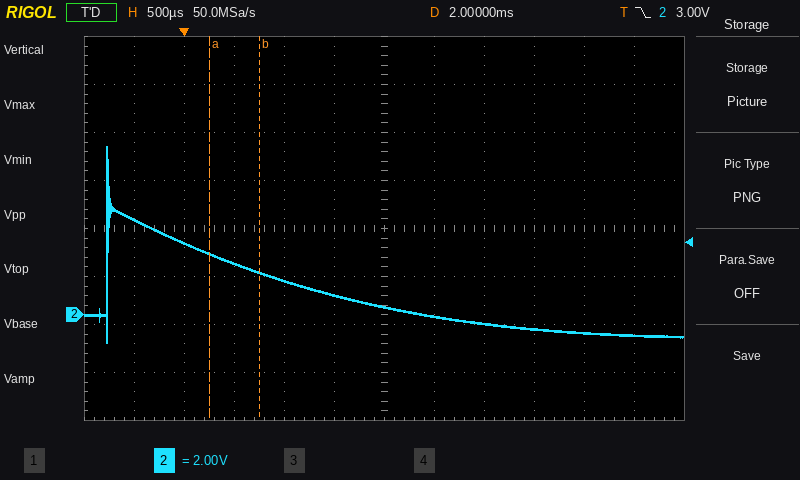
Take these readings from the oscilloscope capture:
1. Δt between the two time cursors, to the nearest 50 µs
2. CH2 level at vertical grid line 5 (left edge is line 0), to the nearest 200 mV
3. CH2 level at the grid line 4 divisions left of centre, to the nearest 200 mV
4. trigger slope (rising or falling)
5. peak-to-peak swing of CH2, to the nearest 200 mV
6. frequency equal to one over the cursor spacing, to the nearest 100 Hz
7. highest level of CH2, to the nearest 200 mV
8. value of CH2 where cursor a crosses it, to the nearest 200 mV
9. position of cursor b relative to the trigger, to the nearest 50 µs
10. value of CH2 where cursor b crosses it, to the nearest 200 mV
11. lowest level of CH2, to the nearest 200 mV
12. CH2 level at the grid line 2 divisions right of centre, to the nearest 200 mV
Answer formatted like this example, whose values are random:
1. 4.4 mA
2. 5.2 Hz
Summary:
1. 500 µs
2. 800 mV
3. 3.0 V
4. falling
5. 8.2 V
6. 2.0 kHz
7. 7.0 V
8. 2.6 V
9. +750 µs
10. 1.8 V
11. -1.2 V
12. -400 mV
